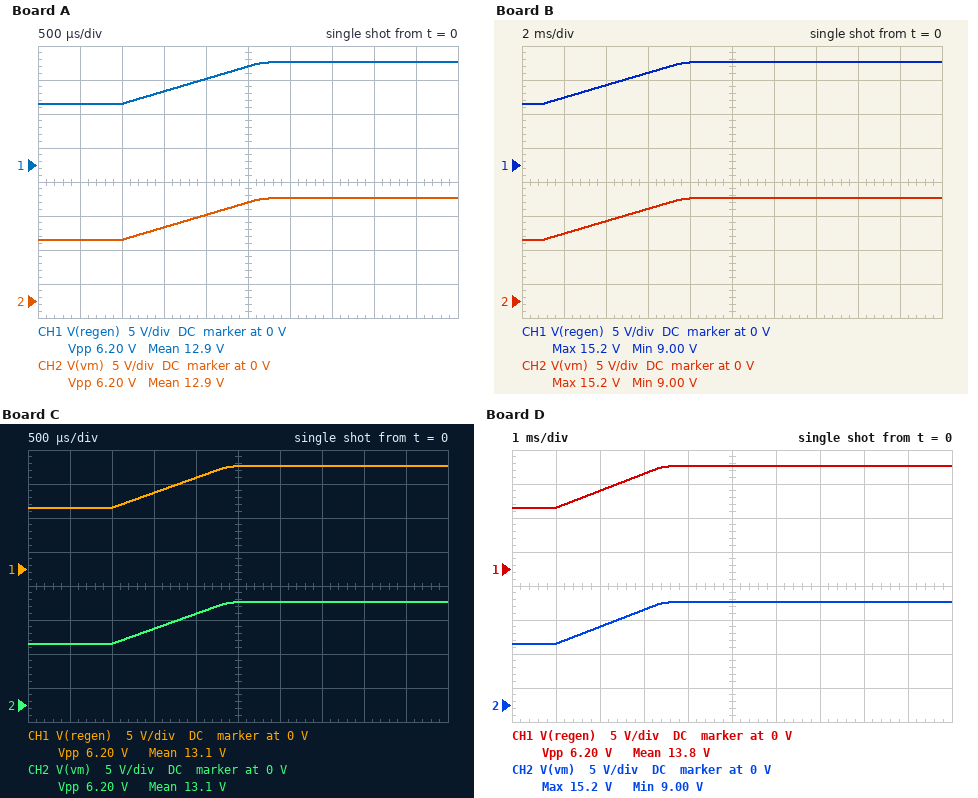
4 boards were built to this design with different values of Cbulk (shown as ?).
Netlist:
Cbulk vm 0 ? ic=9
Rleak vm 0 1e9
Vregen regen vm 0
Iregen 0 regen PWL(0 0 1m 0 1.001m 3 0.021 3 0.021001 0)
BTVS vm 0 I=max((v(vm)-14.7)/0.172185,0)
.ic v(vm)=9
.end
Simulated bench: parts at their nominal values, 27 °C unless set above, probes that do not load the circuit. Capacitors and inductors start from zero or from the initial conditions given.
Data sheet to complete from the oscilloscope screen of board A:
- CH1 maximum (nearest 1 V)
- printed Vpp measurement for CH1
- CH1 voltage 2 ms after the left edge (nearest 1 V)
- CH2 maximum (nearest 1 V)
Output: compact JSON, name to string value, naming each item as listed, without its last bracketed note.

{"CH1 maximum": "15 V", "printed Vpp measurement for CH1": "6.20 V", "CH1 voltage 2 ms after the left edge": "13 V", "CH2 maximum": "15 V"}
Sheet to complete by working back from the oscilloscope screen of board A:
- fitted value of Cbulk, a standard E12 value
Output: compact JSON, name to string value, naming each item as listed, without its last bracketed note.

{"fitted value of Cbulk, a standard E12 value": "820 µF"}
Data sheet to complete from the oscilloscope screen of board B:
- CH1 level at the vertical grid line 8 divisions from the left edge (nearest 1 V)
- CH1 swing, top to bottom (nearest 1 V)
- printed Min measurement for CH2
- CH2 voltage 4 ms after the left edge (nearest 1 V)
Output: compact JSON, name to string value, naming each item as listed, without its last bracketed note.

{"CH1 level at the vertical grid line 8 divisions from the left edge": "15 V", "CH1 swing, top to bottom": "6 V", "printed Min measurement for CH2": "9.00 V", "CH2 voltage 4 ms after the left edge": "12 V"}
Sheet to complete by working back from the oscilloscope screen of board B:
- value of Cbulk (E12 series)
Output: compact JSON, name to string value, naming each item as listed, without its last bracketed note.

{"value of Cbulk": "3.3 mF"}
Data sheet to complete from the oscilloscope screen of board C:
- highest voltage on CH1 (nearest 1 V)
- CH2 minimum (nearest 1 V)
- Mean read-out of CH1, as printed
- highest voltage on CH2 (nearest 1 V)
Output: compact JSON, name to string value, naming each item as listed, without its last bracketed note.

{"highest voltage on CH1": "15 V", "CH2 minimum": "9 V", "Mean read-out of CH1, as printed": "13.1 V", "highest voltage on CH2": "15 V"}
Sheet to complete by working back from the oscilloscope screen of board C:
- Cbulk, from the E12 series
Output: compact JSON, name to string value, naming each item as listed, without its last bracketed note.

{"Cbulk, from the E12 series": "680 µF"}
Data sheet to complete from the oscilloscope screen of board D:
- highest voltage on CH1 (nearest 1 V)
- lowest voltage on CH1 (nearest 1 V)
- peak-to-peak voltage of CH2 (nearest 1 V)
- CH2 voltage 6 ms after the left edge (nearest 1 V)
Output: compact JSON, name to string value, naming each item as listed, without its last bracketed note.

{"highest voltage on CH1": "15 V", "lowest voltage on CH1": "9 V", "peak-to-peak voltage of CH2": "6 V", "CH2 voltage 6 ms after the left edge": "15 V"}
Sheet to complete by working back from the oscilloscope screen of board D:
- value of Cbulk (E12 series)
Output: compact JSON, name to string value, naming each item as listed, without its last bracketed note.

{"value of Cbulk": "1.2 mF"}
